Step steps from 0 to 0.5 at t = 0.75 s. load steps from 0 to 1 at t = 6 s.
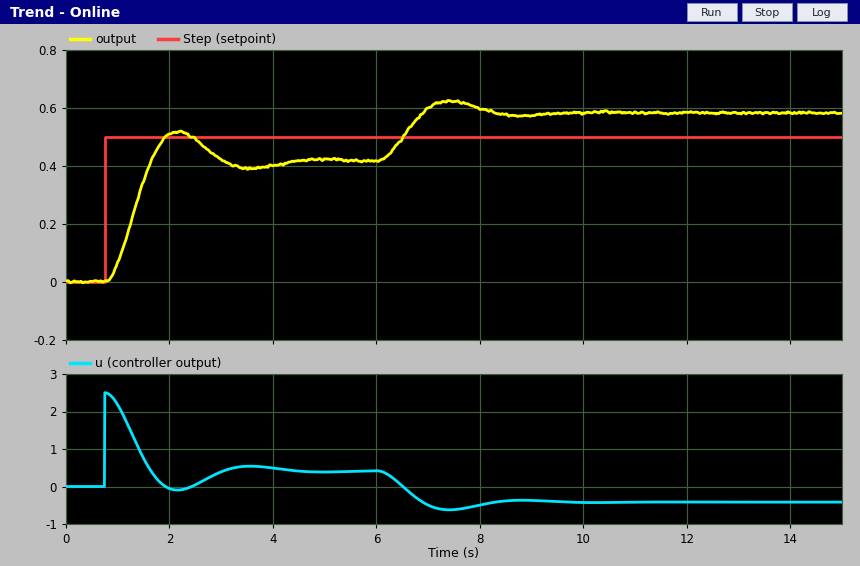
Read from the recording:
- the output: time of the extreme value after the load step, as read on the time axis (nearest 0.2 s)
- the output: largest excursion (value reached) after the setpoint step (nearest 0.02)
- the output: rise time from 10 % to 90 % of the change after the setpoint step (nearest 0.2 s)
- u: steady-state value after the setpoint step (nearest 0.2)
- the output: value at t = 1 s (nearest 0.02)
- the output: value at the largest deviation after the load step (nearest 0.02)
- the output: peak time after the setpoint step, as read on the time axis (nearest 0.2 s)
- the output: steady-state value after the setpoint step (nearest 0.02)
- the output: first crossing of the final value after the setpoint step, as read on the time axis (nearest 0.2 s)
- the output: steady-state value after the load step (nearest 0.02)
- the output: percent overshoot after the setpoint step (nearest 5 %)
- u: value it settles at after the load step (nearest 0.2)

7.4 s
0.52
0.6 s
0.4
0.06
0.62
2.2 s
0.42
1.6 s
0.58
25 %
-0.4
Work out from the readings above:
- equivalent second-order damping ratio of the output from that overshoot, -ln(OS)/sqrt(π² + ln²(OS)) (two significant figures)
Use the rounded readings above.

0.40
